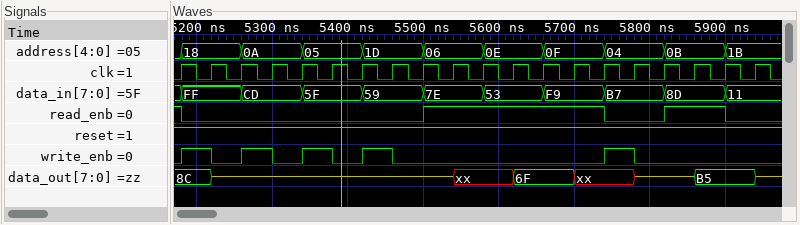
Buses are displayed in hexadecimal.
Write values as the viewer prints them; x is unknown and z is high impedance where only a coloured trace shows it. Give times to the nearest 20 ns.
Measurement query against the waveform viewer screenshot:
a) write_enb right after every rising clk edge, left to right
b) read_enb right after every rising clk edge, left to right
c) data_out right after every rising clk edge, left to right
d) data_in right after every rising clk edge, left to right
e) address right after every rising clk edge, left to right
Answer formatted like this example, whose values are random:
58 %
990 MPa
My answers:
1 0 1 0 1 0 1 0 0 0 0 0 0 0 1 0 0 0 0 0
0 0 0 0 0 0 0 0 1 1 1 1 1 1 0 0 1 1 0 0
8C, z, z, z, z, z, z, z, z, xx, xx, 6F, 6F, xx, xx, z, z, B5, B5, z
FF, FF, CD, CD, 5F, 5F, 59, 59, 7E, 7E, 53, 53, F9, F9, B7, B7, 8D, 8D, 11, 11
18, 18, 0A, 0A, 05, 05, 1D, 1D, 06, 06, 0E, 0E, 0F, 0F, 04, 04, 0B, 0B, 1B, 1B
